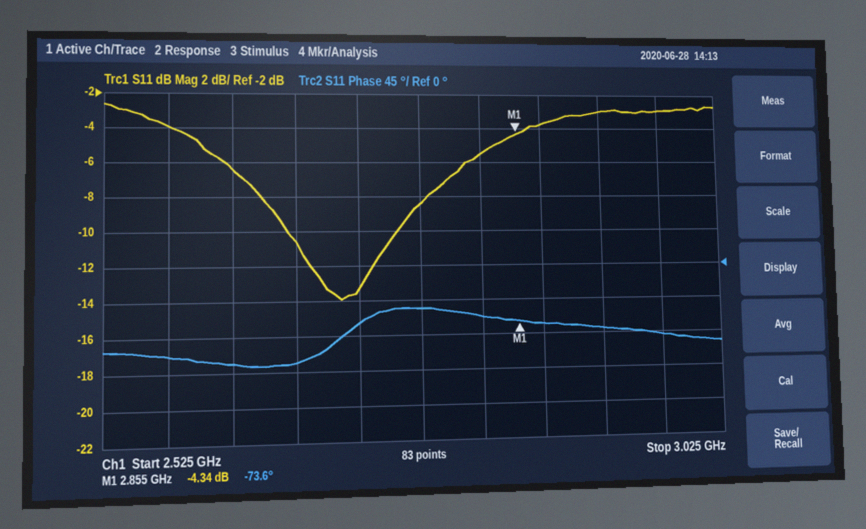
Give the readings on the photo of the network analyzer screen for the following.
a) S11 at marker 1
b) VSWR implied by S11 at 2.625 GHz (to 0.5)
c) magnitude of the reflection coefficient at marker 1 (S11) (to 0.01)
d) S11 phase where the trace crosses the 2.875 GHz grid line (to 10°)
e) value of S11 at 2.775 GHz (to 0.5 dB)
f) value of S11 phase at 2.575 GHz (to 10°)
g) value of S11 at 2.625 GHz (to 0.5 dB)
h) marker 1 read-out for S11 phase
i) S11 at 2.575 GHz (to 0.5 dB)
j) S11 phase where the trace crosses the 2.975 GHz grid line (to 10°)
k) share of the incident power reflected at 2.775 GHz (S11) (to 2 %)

-4.34 dB
3.0
0.61
-80°
-8.5 dB
-110°
-6.5 dB
-73.6°
-4.0 dB
-90°
14 %
